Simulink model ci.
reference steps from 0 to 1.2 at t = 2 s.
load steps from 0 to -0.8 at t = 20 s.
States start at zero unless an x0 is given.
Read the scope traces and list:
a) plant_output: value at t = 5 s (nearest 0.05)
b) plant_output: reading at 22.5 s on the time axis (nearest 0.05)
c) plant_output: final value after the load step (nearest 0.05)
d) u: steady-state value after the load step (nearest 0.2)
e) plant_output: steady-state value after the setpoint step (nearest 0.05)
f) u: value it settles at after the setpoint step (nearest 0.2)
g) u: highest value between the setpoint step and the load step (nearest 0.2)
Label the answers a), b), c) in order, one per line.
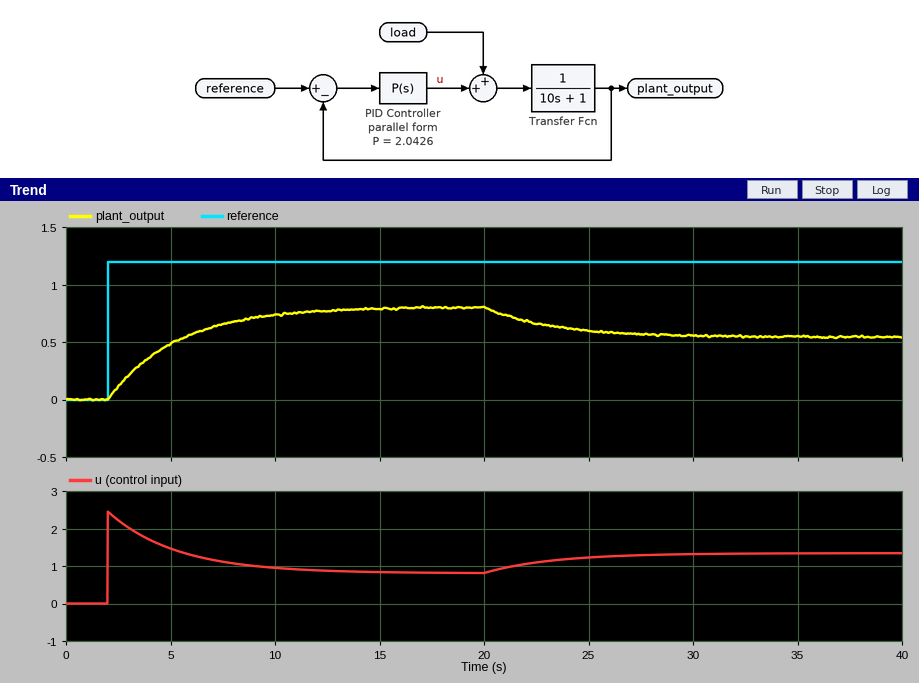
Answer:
a) 0.50
b) 0.65
c) 0.55
d) 1.4
e) 0.80
f) 0.8
g) 2.4
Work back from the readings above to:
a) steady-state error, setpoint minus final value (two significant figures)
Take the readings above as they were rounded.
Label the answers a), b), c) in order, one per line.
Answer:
a) 0.40
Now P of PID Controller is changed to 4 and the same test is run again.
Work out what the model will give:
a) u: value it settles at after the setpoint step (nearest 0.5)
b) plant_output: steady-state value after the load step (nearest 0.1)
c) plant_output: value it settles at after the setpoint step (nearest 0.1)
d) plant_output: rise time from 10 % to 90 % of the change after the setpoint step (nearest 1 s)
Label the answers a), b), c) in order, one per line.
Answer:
a) 1.0
b) 0.8
c) 1.0
d) 4 s
